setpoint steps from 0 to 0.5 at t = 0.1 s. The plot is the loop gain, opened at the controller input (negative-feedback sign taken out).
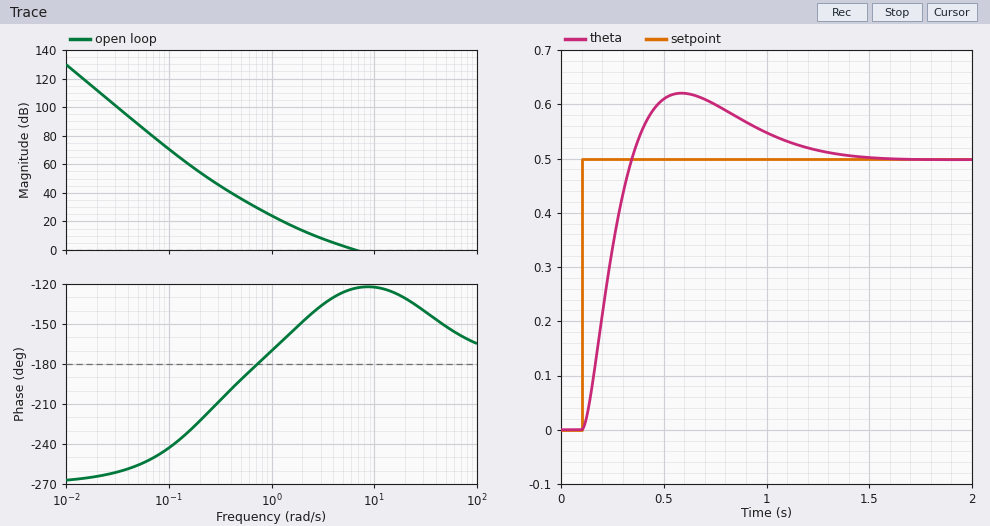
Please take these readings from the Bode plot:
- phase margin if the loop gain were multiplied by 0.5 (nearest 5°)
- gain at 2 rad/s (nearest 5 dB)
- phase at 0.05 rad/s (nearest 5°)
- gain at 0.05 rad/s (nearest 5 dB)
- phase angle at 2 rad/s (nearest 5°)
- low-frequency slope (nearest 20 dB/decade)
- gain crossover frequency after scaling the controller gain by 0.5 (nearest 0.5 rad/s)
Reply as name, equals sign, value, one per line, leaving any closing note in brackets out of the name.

phase margin if the loop gain were multiplied by 0.5 = 50°
gain at 2 rad/s = 15 dB
phase at 0.05 rad/s = -255°
gain at 0.05 rad/s = 90 dB
phase angle at 2 rad/s = -150°
low-frequency slope = -60 dB/decade
gain crossover frequency after scaling the controller gain by 0.5 = 3.5 rad/s
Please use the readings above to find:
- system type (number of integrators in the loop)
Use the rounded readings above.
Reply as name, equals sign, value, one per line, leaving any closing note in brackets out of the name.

system type = 3
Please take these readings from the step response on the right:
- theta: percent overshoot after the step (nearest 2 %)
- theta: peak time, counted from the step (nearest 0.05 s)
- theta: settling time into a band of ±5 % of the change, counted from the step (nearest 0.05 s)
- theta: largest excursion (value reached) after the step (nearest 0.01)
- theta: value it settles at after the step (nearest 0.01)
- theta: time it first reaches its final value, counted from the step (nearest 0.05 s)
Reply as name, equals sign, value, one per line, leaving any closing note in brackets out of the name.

theta: percent overshoot after the step = 24 %
theta: peak time, counted from the step = 0.50 s
theta: settling time into a band of ±5 % of the change, counted from the step = 1.05 s
theta: largest excursion (value reached) after the step = 0.62
theta: value it settles at after the step = 0.50
theta: time it first reaches its final value, counted from the step = 0.25 s
